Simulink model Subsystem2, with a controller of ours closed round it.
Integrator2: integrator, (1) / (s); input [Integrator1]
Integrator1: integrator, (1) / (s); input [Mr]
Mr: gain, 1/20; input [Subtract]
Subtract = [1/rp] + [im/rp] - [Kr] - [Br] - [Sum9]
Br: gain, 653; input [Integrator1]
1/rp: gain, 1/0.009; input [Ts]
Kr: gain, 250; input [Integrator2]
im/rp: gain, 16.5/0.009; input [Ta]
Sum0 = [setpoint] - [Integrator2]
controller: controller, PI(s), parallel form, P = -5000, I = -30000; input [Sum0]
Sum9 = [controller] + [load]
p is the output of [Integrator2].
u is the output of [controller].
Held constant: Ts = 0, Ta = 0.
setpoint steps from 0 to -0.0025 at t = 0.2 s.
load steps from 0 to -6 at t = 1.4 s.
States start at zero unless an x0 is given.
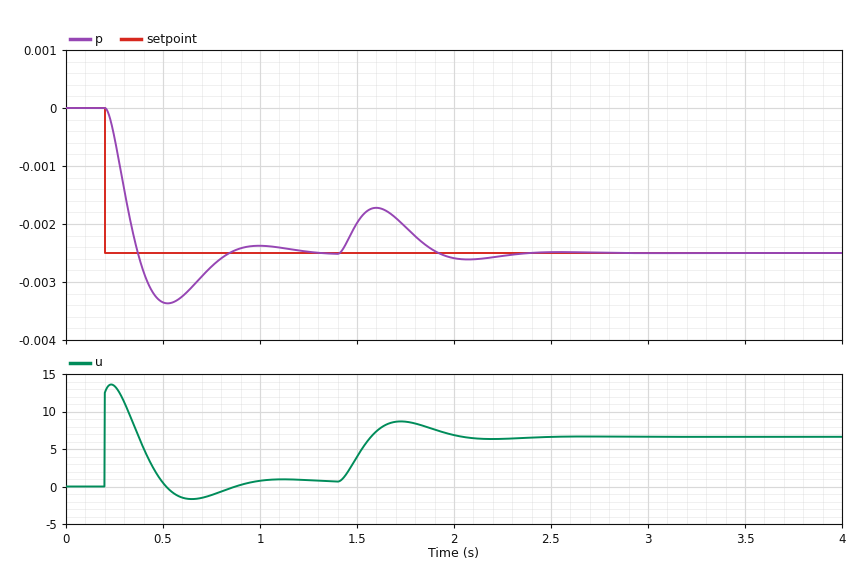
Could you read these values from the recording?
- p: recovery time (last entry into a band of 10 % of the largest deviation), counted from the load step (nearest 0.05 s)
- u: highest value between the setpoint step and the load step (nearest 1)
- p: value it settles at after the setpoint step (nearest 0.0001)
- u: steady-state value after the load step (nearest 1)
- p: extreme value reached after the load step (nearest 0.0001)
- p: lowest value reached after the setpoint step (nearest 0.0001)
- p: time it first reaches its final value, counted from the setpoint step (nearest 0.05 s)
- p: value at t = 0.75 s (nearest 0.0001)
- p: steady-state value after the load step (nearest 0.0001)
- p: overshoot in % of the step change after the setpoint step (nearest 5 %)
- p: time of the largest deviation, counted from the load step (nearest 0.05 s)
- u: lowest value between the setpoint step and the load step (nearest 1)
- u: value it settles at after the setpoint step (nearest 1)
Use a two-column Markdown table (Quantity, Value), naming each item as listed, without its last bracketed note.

| Quantity | Value |
|---|---|
| p: recovery time (last entry into a band of 10 % of the largest deviation), counted from the load step | 0.80 s |
| u: highest value between the setpoint step and the load step | 14 |
| p: value it settles at after the setpoint step | -0.0025 |
| u: steady-state value after the load step | 7 |
| p: extreme value reached after the load step | -0.0017 |
| p: lowest value reached after the setpoint step | -0.0034 |
| p: time it first reaches its final value, counted from the setpoint step | 0.15 s |
| p: value at t = 0.75 s | -0.0027 |
| p: steady-state value after the load step | -0.0025 |
| p: overshoot in % of the step change after the setpoint step | 35 % |
| p: time of the largest deviation, counted from the load step | 0.20 s |
| u: lowest value between the setpoint step and the load step | -2 |
| u: value it settles at after the setpoint step | 1 |
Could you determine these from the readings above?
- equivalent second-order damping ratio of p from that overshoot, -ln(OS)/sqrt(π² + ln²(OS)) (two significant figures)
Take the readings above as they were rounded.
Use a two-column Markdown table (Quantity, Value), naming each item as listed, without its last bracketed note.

| Quantity | Value |
|---|---|
| equivalent second-order damping ratio of p from that overshoot, -ln(OS)/sqrt(π² + ln²(OS)) | 0.32 |
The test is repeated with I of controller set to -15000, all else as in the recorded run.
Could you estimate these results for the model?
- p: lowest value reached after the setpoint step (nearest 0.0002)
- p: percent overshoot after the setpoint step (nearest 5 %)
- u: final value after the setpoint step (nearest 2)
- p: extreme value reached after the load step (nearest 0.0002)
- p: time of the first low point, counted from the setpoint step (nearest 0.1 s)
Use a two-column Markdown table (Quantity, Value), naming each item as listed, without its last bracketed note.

| Quantity | Value |
|---|---|
| p: lowest value reached after the setpoint step | -0.0030 |
| p: percent overshoot after the setpoint step | 20 % |
| u: final value after the setpoint step | 0 |
| p: extreme value reached after the load step | -0.0016 |
| p: time of the first low point, counted from the setpoint step | 0.4 s |
